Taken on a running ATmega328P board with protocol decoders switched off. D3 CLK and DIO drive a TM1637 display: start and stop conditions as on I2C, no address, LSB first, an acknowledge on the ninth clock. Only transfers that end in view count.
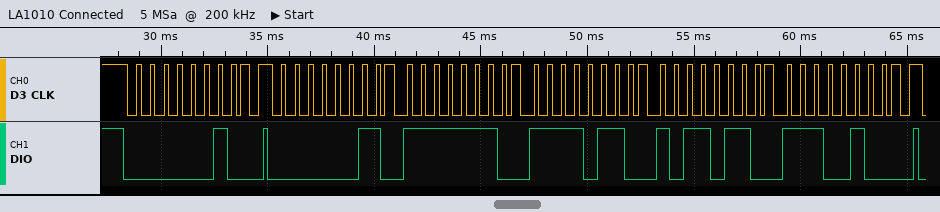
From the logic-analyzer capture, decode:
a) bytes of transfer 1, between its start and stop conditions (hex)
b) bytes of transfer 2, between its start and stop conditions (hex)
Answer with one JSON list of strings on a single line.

["40", "C0 7F 6F 6D 27"]
